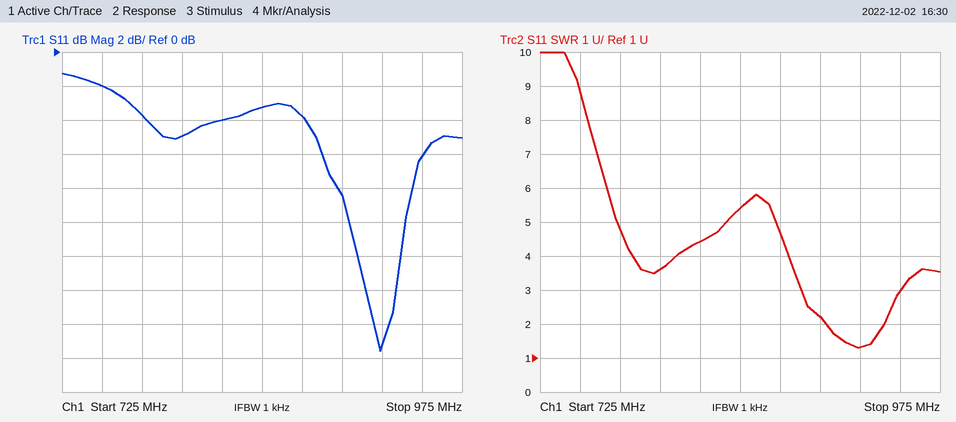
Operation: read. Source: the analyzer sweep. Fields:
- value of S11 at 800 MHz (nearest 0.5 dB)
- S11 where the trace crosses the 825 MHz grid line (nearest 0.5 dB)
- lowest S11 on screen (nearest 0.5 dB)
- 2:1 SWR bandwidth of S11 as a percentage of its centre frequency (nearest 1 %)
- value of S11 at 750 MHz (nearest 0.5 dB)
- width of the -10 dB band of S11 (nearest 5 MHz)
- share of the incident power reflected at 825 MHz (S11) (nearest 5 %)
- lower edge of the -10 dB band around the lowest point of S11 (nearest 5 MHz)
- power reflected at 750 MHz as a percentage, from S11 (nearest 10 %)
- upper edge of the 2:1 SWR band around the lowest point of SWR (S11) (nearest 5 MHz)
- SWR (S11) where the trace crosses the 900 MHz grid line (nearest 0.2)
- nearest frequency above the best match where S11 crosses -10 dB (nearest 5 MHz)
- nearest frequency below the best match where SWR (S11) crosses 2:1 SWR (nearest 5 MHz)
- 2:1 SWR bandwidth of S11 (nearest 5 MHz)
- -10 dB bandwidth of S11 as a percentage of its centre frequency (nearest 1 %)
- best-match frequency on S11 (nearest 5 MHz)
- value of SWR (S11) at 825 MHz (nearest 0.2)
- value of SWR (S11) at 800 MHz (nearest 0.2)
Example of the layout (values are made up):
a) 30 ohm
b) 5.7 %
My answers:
a) -5.0 dB
b) -4.0 dB
c) -17.5 dB
d) 4 %
e) -2.0 dB
f) 35 MHz
g) 40 %
h) 905 MHz
i) 60 %
j) 940 MHz
k) 2.2
l) 940 MHz
m) 905 MHz
n) 35 MHz
o) 4 %
p) 925 MHz
q) 4.4
r) 3.6
